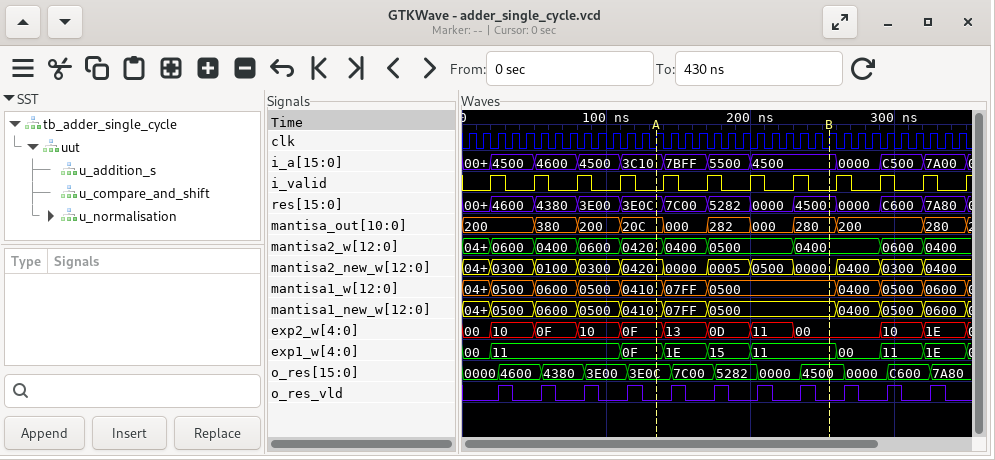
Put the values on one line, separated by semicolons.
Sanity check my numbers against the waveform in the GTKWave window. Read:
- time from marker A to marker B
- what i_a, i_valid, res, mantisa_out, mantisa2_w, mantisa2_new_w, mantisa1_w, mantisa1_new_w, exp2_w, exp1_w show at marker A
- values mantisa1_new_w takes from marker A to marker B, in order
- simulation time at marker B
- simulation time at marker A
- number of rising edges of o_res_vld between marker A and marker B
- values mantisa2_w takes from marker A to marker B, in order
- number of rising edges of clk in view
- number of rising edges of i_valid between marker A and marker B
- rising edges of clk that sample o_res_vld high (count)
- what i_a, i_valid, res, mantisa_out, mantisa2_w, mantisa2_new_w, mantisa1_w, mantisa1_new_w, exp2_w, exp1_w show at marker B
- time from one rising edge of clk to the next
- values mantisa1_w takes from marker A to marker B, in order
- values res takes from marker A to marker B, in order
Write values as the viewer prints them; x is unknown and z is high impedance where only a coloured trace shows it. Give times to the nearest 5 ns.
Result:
120 ns; i_a=3C10, i_valid=0, res=3E0C, mantisa_out=20C, mantisa2_w=0420, mantisa2_new_w=0420, mantisa1_w=0410, mantisa1_new_w=0410, exp2_w=0F, exp1_w=0F; 0410, 07FF, 0500; 255 ns; 135 ns; 4; 0420, 0400, 0500, 0400; 35; 4; 11; i_a=4500, i_valid=0, res=4500, mantisa_out=280, mantisa2_w=0400, mantisa2_new_w=0000, mantisa1_w=0500, mantisa1_new_w=0500, exp2_w=00, exp1_w=11; 10 ns; 0410, 07FF, 0500; 3E0C, 7C00, 5282, 0000, 4500
